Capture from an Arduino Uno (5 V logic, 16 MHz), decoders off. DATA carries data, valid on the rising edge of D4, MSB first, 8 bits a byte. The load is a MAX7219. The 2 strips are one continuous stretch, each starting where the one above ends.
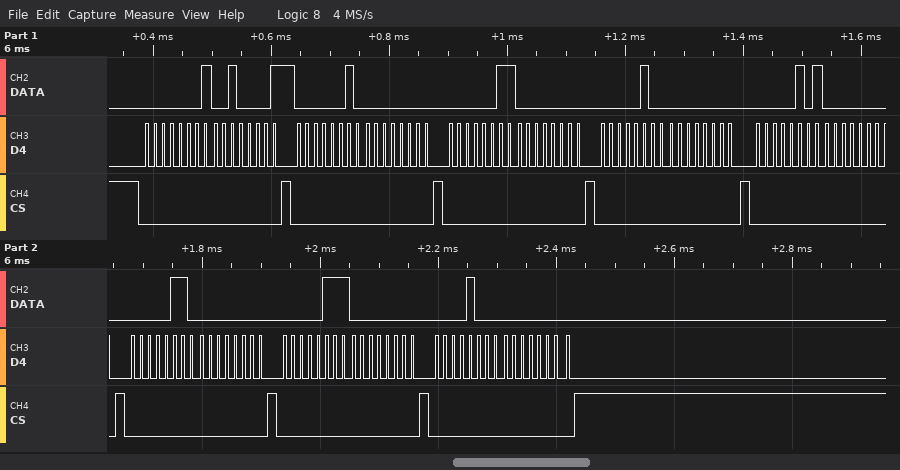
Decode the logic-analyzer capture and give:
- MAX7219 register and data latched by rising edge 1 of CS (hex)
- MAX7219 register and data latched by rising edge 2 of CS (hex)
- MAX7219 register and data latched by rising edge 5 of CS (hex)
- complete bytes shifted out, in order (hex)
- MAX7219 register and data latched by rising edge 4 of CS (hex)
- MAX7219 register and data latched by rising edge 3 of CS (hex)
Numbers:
register 0x1, data 0x21
register 0x2, data 0x00
register 0x5, data 0x00
0x01 0x21 0x02 0x00 0x03 0x00 0x04 0x00 0x05 0x00 0x06 0x00 0x07 0x00 0x08 0x00
register 0x4, data 0x00
register 0x3, data 0x00
